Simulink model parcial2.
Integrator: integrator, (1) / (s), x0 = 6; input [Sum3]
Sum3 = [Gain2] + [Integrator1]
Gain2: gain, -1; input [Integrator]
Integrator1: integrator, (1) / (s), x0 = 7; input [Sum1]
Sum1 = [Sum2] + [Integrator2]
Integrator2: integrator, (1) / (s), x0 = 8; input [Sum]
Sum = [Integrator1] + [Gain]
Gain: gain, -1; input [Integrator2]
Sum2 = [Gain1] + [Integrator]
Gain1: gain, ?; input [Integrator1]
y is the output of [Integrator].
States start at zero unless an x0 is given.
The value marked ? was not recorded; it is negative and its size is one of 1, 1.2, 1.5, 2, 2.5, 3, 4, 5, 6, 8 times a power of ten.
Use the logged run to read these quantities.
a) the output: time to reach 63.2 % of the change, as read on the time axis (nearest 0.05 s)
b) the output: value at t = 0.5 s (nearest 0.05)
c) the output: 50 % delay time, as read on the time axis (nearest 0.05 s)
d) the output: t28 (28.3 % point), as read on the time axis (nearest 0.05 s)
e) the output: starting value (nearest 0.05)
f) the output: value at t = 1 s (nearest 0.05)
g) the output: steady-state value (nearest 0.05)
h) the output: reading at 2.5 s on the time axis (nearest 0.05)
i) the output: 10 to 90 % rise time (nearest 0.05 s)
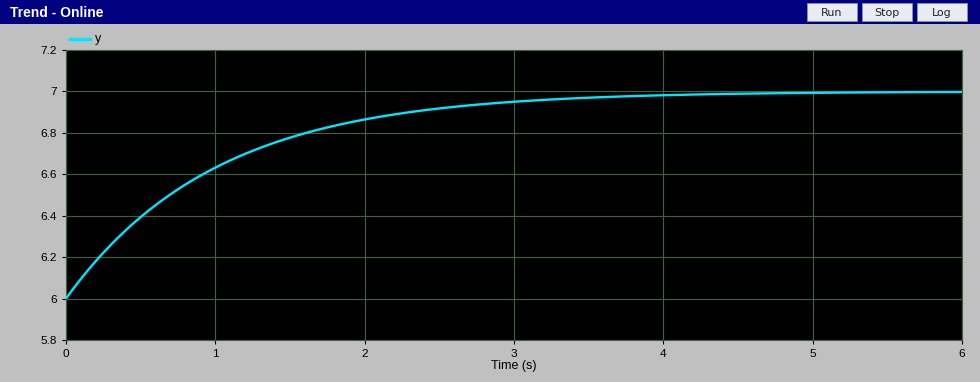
1.00 s
6.40
0.70 s
0.35 s
6.00
6.65
7.00
6.90
2.20 s
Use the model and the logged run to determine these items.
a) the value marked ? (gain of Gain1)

-2
